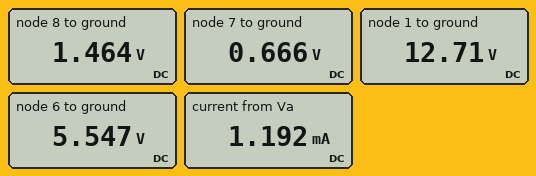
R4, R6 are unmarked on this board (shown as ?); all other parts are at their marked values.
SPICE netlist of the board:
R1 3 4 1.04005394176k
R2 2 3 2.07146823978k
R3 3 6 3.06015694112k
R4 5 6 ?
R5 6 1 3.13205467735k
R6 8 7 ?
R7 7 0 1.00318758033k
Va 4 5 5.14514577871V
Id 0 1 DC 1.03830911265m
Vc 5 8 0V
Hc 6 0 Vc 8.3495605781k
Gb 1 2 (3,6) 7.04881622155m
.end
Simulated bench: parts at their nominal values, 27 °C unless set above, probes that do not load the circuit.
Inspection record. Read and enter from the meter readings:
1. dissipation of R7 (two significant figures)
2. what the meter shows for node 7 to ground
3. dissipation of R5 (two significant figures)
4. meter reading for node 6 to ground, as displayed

440 µW
0.666 V
16 mW
5.547 V
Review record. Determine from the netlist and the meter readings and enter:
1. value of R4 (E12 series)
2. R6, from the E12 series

2.2 kΩ
1.2 kΩ
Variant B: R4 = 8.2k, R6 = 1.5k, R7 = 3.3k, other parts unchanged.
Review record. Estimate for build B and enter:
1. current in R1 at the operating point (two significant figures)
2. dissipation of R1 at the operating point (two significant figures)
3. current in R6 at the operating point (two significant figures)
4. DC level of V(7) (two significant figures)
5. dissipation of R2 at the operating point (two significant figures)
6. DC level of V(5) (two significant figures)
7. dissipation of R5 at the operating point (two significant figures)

960 µA
960 µW
1.7 mA
5.6 V
2.1 mW
8.1 V
3.4 µW
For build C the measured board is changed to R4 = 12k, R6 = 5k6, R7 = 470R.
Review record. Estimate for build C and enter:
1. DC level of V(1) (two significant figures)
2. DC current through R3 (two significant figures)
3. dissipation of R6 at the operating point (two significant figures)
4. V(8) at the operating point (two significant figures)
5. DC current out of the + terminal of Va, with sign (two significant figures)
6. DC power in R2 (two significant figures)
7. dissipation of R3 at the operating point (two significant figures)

22 V
130 µA
61 mW
20 V
-2.7 mA
16 mW
52 µW
